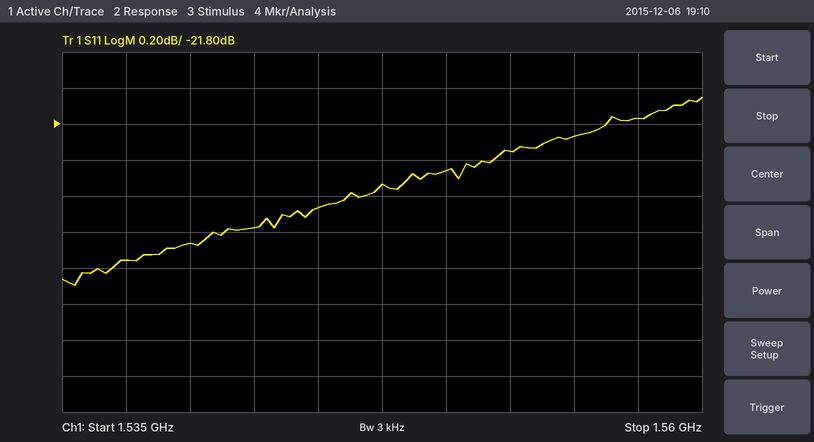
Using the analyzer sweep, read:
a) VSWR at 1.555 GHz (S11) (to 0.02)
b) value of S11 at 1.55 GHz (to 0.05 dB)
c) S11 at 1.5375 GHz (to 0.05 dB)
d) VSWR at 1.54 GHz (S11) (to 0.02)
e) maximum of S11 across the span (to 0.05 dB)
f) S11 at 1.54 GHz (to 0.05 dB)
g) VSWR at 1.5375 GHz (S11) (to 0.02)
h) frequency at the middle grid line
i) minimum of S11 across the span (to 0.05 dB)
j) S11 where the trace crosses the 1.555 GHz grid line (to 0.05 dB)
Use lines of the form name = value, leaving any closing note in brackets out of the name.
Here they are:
VSWR at 1.555 GHz (S11) = 1.18
value of S11 at 1.55 GHz = -22.05 dB
S11 at 1.5375 GHz = -22.55 dB
VSWR at 1.54 GHz (S11) = 1.16
maximum of S11 across the span = -21.65 dB
S11 at 1.54 GHz = -22.45 dB
VSWR at 1.5375 GHz (S11) = 1.16
frequency at the middle grid line = 1.5475 GHz
minimum of S11 across the span = -22.70 dB
S11 where the trace crosses the 1.555 GHz grid line = -21.85 dB
